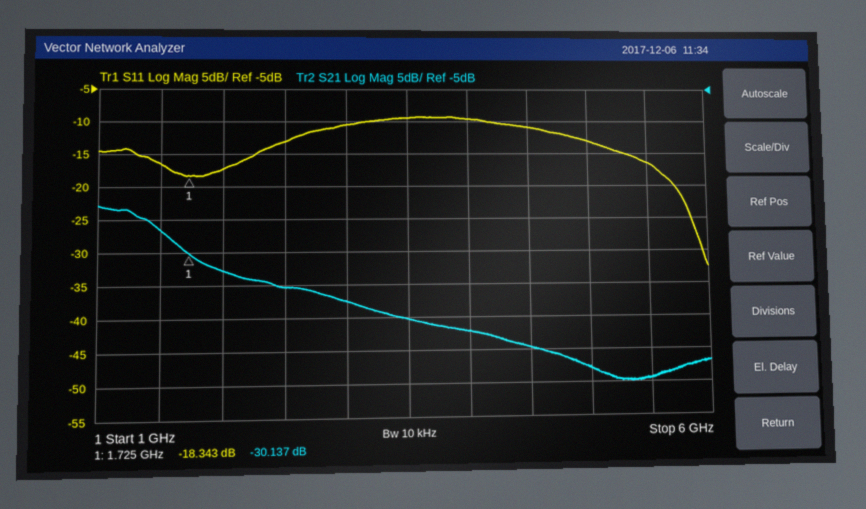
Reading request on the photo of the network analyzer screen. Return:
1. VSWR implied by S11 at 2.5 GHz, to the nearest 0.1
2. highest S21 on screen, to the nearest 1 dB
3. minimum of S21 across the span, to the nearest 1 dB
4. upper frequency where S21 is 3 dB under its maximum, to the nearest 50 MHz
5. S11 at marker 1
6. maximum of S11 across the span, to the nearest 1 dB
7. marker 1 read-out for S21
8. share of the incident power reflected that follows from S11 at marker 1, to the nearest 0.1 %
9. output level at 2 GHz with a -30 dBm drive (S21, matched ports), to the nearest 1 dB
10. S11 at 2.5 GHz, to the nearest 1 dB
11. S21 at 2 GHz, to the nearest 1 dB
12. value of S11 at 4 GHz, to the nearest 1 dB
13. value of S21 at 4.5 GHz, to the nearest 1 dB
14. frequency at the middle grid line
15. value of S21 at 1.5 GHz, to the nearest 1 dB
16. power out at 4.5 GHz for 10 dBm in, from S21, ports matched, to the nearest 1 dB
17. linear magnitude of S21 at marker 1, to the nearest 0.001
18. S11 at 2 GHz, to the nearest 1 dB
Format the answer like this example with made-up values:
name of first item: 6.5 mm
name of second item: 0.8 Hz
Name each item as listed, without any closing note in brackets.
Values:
VSWR implied by S11 at 2.5 GHz, to the nearest 0.1: 1.6
highest S21 on screen, to the nearest 1 dB: -23 dB
minimum of S21 across the span, to the nearest 1 dB: -50 dB
upper frequency where S21 is 3 dB under its maximum, to the nearest 50 MHz: 1.45 GHz
S11 at marker 1: -18.343 dB
maximum of S11 across the span, to the nearest 1 dB: -9 dB
marker 1 read-out for S21: -30.137 dB
share of the incident power reflected that follows from S11 at marker 1, to the nearest 0.1 %: 1.5 %
output level at 2 GHz with a -30 dBm drive (S21, matched ports), to the nearest 1 dB: -63 dBm
S11 at 2.5 GHz, to the nearest 1 dB: -13 dB
S21 at 2 GHz, to the nearest 1 dB: -33 dB
value of S11 at 4 GHz, to the nearest 1 dB: -10 dB
value of S21 at 4.5 GHz, to the nearest 1 dB: -45 dB
frequency at the middle grid line: 3.5 GHz
value of S21 at 1.5 GHz, to the nearest 1 dB: -27 dB
power out at 4.5 GHz for 10 dBm in, from S21, ports matched, to the nearest 1 dB: -35 dBm
linear magnitude of S21 at marker 1, to the nearest 0.001: 0.031
S11 at 2 GHz, to the nearest 1 dB: -17 dB
